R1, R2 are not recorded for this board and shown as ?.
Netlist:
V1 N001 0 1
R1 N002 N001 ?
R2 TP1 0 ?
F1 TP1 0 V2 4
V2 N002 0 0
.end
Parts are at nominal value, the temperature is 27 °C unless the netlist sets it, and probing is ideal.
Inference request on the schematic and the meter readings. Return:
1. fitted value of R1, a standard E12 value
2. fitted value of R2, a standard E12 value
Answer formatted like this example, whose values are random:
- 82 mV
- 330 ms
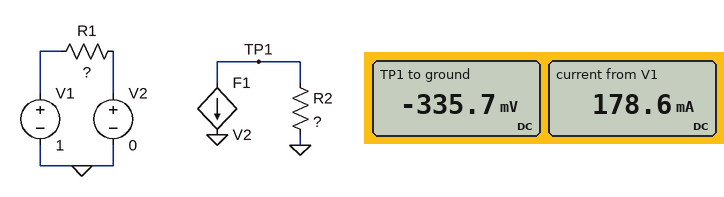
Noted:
- 5.6 Ω
- 0.47 Ω
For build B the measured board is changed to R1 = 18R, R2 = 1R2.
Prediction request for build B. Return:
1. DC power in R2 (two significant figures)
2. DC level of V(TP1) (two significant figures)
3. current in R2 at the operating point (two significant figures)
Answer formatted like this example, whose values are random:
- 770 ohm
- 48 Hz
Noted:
- 59 mW
- -270 mV
- 220 mA
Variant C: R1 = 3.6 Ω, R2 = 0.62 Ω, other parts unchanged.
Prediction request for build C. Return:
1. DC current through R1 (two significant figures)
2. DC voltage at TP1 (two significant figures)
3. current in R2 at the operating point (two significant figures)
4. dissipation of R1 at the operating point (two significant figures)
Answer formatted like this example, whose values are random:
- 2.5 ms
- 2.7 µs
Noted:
- 280 mA
- -690 mV
- 1.1 A
- 280 mW
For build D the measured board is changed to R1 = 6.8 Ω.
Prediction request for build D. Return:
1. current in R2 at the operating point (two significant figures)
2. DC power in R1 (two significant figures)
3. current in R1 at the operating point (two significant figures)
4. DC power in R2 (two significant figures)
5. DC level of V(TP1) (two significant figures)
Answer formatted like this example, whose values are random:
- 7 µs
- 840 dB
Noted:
- 590 mA
- 150 mW
- 150 mA
- 160 mW
- -280 mV
